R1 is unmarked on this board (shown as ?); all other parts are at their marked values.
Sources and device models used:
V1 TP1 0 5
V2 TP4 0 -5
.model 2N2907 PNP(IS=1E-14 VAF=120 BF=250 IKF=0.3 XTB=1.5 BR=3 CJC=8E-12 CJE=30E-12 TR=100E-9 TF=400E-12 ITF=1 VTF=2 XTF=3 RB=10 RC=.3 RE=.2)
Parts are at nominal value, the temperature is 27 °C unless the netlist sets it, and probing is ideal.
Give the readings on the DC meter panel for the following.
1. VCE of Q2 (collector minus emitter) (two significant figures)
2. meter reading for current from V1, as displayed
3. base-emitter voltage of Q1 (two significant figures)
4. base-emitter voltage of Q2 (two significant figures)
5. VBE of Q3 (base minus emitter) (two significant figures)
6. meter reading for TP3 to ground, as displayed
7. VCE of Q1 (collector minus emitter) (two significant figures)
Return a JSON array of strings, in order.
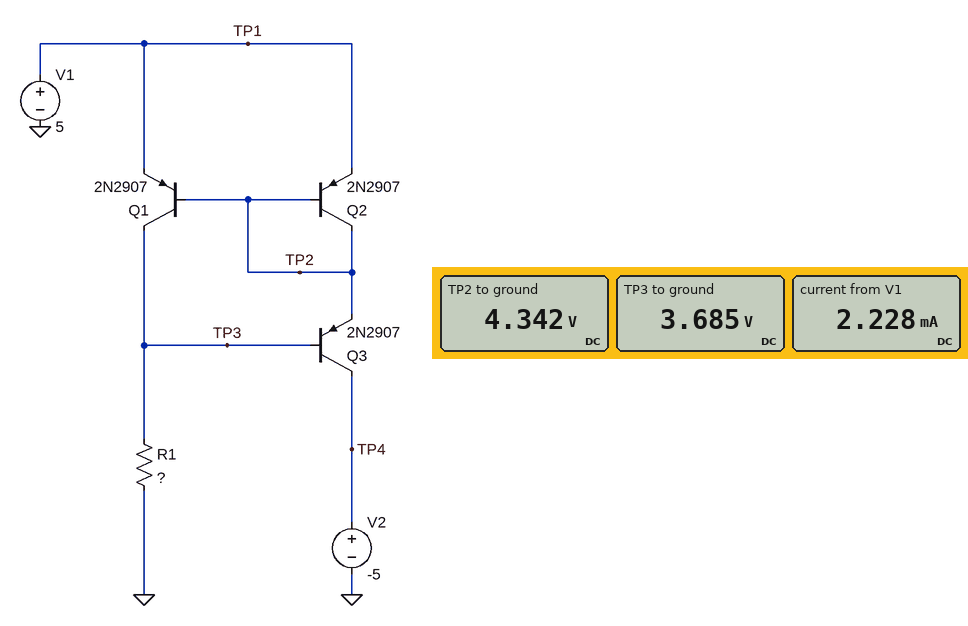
["-660 mV", "2.228 mA", "-660 mV", "-660 mV", "-660 mV", "3.685 V", "-1.3 V"]
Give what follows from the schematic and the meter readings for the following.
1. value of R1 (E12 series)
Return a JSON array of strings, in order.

["3.3 kΩ"]
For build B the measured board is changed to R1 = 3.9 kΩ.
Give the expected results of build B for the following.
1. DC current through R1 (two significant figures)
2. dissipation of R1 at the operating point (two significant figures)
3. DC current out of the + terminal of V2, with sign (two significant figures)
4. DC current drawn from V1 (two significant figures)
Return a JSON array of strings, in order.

["950 µA", "3.5 mW", "-940 µA", "1.9 mA"]
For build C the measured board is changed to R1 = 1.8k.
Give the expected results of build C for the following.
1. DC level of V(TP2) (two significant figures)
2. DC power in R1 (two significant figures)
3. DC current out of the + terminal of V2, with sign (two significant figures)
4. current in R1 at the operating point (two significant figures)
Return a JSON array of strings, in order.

["4.3 V", "7.4 mW", "-2.0 mA", "2.0 mA"]
